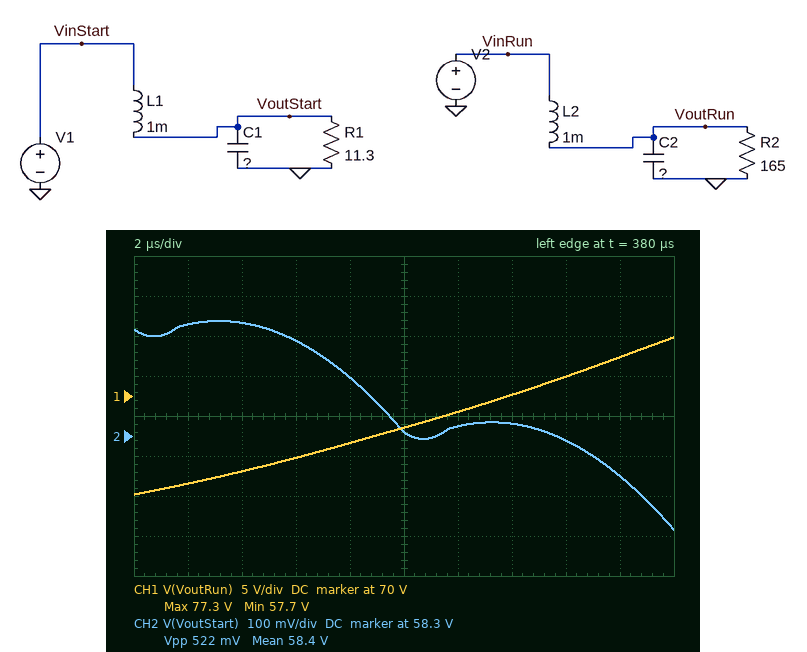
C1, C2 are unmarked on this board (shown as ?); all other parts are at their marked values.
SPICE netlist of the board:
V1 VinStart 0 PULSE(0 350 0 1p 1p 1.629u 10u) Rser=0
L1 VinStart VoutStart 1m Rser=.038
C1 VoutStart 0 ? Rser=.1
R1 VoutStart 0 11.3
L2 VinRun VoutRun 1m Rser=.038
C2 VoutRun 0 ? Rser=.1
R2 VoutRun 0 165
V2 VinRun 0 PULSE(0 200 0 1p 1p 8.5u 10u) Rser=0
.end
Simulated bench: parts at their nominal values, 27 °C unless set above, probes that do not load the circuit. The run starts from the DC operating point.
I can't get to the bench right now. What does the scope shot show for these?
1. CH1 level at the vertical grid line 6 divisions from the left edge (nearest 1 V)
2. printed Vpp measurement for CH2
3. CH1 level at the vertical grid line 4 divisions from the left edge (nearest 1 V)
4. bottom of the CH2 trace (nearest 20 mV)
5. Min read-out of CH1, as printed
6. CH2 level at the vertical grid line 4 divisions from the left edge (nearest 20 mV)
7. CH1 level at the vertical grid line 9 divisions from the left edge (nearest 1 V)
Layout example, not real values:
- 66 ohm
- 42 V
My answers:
- 68 V
- 522 mV
- 64 V
- 58.06 V
- 57.7 V
- 58.44 V
- 75 V
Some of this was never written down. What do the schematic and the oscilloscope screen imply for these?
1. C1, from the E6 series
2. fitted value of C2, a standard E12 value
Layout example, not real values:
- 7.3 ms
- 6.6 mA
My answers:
- 4.7 µF
- 3.3 µF
